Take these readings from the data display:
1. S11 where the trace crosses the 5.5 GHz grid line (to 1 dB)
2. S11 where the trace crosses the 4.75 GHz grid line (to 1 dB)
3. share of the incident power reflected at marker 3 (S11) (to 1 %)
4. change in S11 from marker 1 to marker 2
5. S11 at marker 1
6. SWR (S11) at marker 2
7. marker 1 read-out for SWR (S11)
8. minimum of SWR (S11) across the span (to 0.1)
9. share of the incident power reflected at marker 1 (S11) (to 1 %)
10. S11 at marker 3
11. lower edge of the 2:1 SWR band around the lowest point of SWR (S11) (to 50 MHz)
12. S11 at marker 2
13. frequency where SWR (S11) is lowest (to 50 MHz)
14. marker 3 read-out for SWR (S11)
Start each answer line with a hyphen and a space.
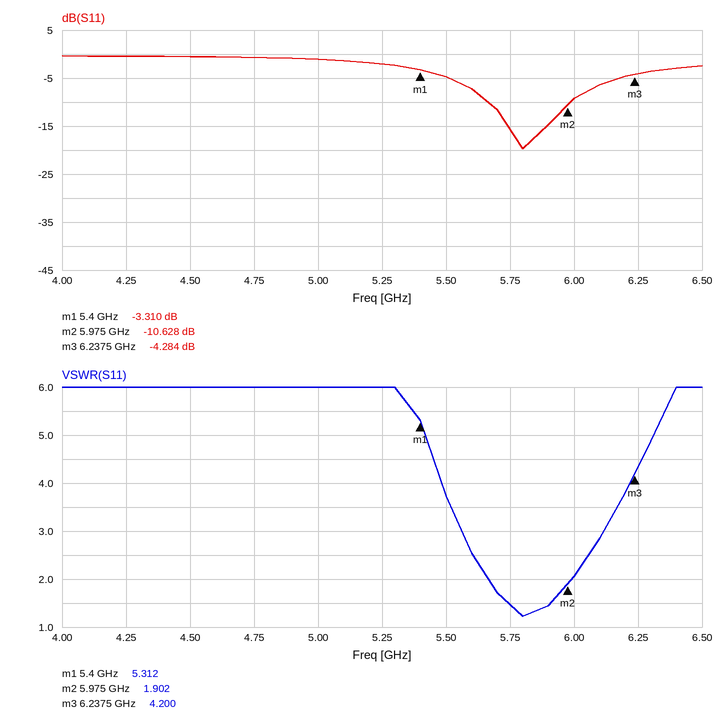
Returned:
- -5 dB
- -1 dB
- 37 %
- -7.318 dB
- -3.310 dB
- 1.902
- 5.312
- 1.2
- 47 %
- -4.284 dB
- 5.65 GHz
- -10.628 dB
- 5.80 GHz
- 4.200
